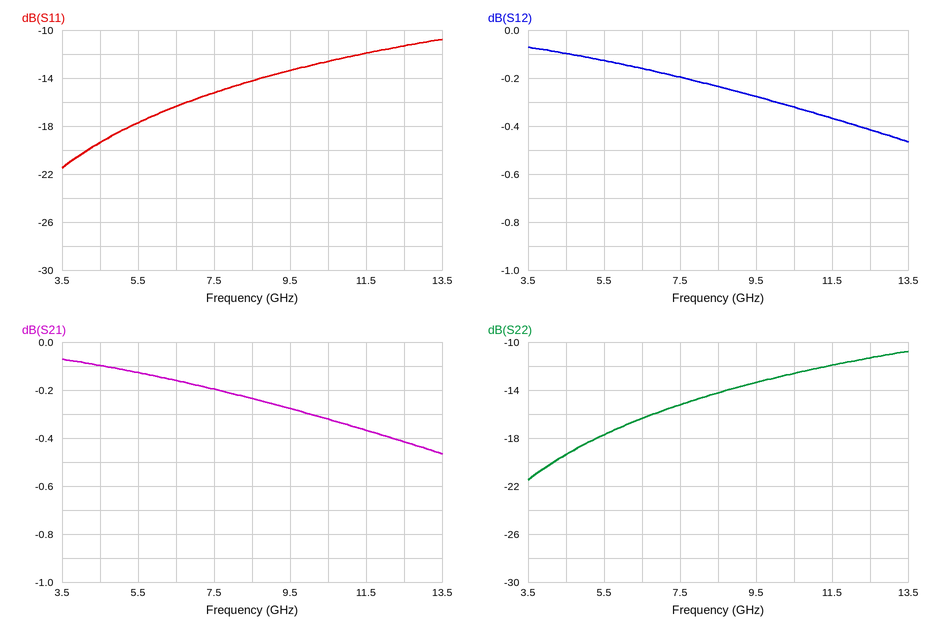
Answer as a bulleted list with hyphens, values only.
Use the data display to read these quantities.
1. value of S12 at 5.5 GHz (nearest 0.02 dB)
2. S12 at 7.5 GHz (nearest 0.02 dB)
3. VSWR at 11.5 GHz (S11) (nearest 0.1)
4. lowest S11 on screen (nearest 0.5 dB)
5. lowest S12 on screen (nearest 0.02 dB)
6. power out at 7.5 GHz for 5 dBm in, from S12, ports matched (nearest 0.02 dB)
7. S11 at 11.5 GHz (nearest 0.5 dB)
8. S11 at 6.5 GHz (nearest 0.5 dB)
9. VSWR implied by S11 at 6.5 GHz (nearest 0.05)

- -0.12 dB
- -0.20 dB
- 1.7
- -21.5 dB
- -0.46 dB
- 4.80 dBm
- -12.0 dB
- -16.5 dB
- 1.35
